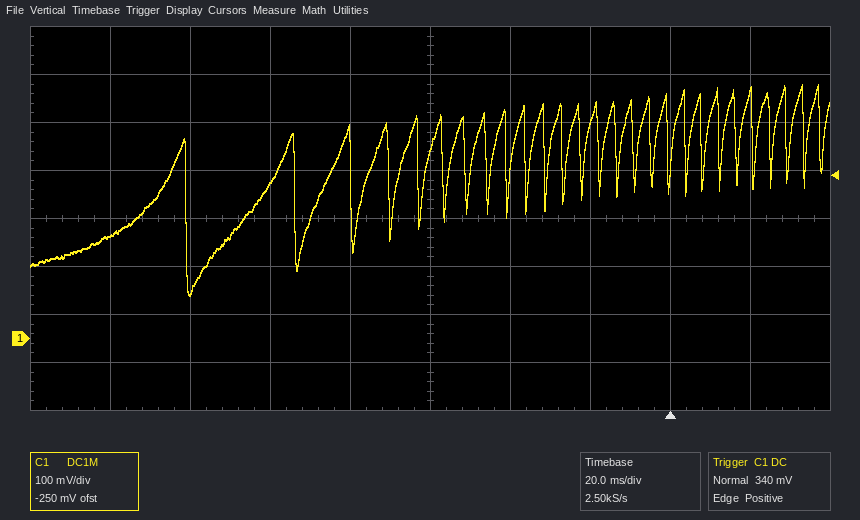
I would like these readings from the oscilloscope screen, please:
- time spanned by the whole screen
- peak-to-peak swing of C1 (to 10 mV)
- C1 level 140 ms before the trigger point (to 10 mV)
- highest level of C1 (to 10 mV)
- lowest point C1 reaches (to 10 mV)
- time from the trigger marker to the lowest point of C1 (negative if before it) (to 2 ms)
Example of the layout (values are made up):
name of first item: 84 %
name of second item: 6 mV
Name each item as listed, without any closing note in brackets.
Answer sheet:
time spanned by the whole screen: 200 ms
peak-to-peak swing of C1: 440 mV
C1 level 140 ms before the trigger point: 210 mV
highest level of C1: 530 mV
lowest point C1 reaches: 90 mV
time from the trigger marker to the lowest point of C1 (negative if before it): -120 ms
